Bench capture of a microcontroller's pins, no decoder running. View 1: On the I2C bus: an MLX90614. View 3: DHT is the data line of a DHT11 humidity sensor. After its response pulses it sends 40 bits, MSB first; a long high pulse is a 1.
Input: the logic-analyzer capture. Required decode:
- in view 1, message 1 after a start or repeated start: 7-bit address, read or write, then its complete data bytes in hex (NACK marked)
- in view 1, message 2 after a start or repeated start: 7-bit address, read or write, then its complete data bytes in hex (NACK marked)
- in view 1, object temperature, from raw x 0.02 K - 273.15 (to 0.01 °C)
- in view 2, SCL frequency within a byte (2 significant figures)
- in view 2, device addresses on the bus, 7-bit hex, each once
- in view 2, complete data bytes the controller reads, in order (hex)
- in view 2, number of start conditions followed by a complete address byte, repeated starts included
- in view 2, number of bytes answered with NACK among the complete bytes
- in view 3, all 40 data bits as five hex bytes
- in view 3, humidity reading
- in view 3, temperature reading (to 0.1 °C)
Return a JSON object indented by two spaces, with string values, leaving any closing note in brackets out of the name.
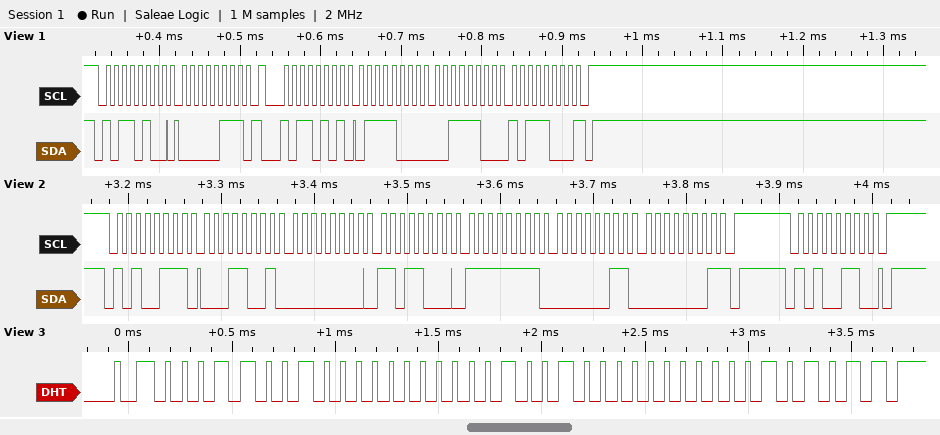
{
  "in view 1, message 1 after a start or repeated start: 7-bit address, read or write, then its complete data bytes in hex": "0x5A write: 07",
  "in view 1, message 2 after a start or repeated start: 7-bit address, read or write, then its complete data bytes in hex": "0x5A read: 78 3C B8 NACK",
  "in view 1, object temperature, from raw x 0.02 K - 273.15": "36.45 °C",
  "in view 2, SCL frequency within a byte": "100 kHz",
  "in view 2, device addresses on the bus, 7-bit hex, each once": "0x53",
  "in view 2, complete data bytes the controller reads, in order": "19 00 D8 FF 03 01",
  "in view 2, number of start conditions followed by a complete address byte, repeated starts included": "2",
  "in view 2, number of bytes answered with NACK among the complete bytes": "1",
  "in view 3, all 40 data bits as five hex bytes": "19 00 12 00 2B",
  "in view 3, humidity reading": "25 %",
  "in view 3, temperature reading": "18.0 °C"
}
